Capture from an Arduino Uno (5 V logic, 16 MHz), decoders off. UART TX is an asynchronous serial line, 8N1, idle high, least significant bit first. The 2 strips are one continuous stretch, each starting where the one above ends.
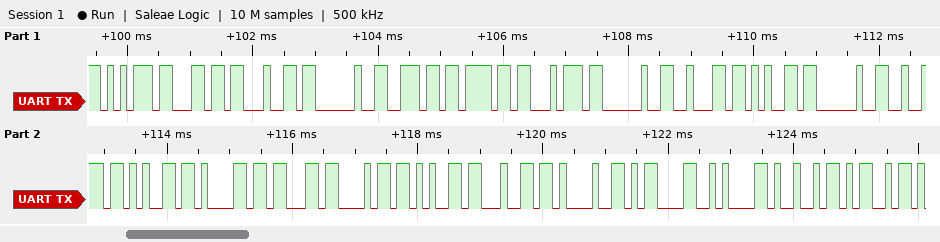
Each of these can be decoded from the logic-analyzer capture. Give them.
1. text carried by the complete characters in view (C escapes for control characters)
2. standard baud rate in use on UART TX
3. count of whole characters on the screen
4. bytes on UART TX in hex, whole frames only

"uld not be reached!\r\nIM"
9600 baud
23
75 6C 64 20 6E 6F 74 20 62 65 20 72 65 61 63 68 65 64 21 0D 0A 49 4D
